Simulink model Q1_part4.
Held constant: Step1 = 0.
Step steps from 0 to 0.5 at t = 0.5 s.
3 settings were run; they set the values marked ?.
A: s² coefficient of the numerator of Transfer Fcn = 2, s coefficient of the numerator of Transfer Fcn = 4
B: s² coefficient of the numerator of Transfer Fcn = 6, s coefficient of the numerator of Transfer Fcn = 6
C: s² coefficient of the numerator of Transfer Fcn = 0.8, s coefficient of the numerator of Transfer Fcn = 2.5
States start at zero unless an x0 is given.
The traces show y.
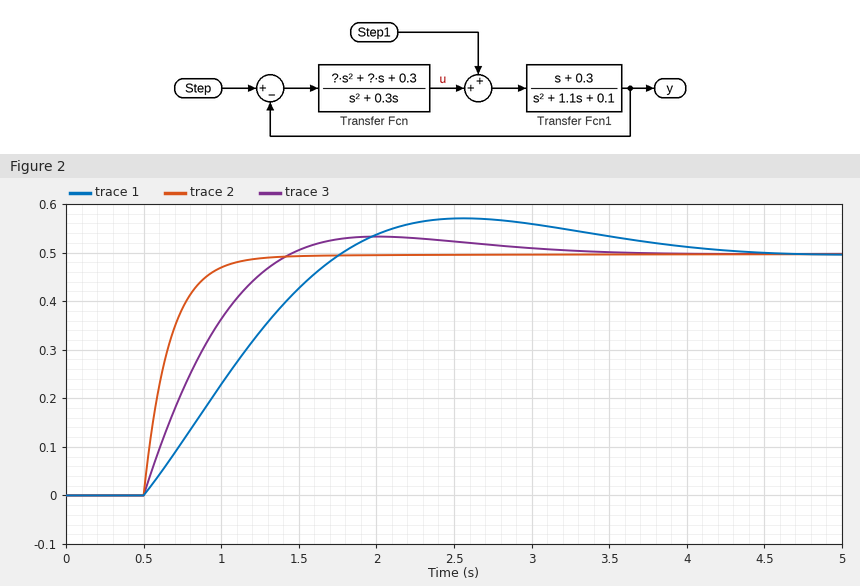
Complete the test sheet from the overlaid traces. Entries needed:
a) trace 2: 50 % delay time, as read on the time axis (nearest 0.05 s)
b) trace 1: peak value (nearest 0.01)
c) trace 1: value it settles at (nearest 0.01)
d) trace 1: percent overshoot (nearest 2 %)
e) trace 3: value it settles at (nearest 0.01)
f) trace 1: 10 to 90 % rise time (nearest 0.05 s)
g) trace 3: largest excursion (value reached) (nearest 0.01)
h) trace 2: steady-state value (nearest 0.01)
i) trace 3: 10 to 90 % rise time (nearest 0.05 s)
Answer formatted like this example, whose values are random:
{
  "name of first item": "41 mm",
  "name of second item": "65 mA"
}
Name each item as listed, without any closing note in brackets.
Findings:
{
  "trace 2: 50 % delay time, as read on the time axis": "0.60 s",
  "trace 1: peak value": "0.57",
  "trace 1: value it settles at": "0.50",
  "trace 1: percent overshoot": "14 %",
  "trace 3: value it settles at": "0.50",
  "trace 1: 10 to 90 % rise time": "0.95 s",
  "trace 3: largest excursion (value reached)": "0.53",
  "trace 2: steady-state value": "0.50",
  "trace 3: 10 to 90 % rise time": "0.70 s"
}
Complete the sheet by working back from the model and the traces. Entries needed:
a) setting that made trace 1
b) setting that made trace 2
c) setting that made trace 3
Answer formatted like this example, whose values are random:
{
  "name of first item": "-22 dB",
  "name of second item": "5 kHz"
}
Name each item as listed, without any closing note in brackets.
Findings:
{
  "setting that made trace 1": "C",
  "setting that made trace 2": "B",
  "setting that made trace 3": "A"
}
